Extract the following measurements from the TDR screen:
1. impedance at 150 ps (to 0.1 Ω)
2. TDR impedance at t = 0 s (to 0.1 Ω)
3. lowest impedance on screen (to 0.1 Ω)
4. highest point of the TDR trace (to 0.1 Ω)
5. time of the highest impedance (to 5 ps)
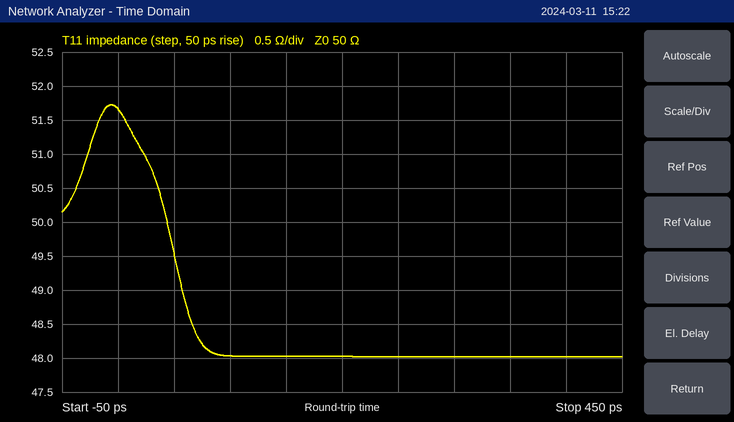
48.0 Ω
51.7 Ω
48.0 Ω
51.7 Ω
-5 ps
